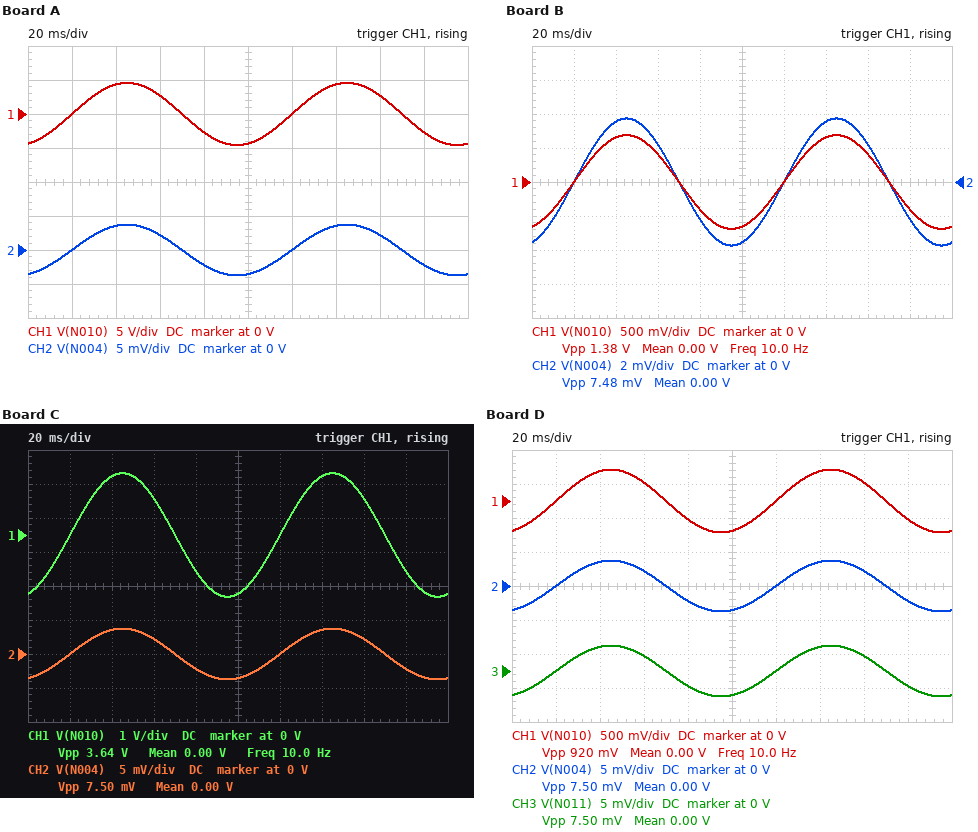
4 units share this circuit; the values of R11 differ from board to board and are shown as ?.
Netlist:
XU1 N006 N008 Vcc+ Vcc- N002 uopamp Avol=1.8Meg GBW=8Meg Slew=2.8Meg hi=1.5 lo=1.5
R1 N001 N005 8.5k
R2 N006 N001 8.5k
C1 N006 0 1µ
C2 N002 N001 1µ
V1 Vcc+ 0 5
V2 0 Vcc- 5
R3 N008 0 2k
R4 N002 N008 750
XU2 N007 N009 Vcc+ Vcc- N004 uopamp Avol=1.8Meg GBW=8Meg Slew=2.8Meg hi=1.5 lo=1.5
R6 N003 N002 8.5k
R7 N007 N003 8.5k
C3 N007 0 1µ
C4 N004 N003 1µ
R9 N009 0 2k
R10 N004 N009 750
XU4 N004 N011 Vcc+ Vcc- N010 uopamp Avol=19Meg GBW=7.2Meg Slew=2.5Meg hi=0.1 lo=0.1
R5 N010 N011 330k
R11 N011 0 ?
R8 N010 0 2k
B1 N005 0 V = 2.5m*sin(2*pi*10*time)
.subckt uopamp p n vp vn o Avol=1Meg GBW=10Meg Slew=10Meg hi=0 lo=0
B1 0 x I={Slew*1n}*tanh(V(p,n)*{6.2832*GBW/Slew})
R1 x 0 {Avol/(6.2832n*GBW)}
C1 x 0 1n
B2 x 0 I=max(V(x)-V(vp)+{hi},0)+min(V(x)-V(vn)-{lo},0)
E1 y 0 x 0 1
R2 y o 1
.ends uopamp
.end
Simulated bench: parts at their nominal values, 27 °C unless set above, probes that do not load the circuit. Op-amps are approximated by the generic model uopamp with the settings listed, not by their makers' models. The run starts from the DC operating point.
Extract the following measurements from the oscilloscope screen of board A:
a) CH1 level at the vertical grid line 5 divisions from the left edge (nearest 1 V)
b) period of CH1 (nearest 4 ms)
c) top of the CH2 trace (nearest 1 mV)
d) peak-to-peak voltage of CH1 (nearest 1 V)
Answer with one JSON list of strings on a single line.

["-4 V", "100 ms", "4 mV", "9 V"]
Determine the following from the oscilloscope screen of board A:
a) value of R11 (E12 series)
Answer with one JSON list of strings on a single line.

["270 Ω"]
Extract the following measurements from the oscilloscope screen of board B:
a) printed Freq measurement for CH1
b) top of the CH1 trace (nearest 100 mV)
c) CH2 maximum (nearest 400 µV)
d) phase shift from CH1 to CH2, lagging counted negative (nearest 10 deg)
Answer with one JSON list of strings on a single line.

["10.0 Hz", "700 mV", "3.6 mV", "0 deg"]
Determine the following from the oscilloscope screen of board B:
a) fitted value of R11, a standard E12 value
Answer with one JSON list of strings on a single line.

["1.8 kΩ"]
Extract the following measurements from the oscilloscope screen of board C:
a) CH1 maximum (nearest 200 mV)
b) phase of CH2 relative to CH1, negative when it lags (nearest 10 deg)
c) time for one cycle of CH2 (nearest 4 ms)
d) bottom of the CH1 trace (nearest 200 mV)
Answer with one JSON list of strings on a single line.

["1.8 V", "0 deg", "100 ms", "-1.8 V"]
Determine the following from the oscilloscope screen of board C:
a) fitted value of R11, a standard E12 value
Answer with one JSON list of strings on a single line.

["680 Ω"]
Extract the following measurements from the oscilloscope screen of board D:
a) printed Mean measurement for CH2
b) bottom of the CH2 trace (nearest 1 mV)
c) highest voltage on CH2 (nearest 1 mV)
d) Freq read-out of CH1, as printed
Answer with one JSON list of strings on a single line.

["0.00 V", "-4 mV", "4 mV", "10.0 Hz"]
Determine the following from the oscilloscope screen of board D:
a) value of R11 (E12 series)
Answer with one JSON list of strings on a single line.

["2.7 kΩ"]
